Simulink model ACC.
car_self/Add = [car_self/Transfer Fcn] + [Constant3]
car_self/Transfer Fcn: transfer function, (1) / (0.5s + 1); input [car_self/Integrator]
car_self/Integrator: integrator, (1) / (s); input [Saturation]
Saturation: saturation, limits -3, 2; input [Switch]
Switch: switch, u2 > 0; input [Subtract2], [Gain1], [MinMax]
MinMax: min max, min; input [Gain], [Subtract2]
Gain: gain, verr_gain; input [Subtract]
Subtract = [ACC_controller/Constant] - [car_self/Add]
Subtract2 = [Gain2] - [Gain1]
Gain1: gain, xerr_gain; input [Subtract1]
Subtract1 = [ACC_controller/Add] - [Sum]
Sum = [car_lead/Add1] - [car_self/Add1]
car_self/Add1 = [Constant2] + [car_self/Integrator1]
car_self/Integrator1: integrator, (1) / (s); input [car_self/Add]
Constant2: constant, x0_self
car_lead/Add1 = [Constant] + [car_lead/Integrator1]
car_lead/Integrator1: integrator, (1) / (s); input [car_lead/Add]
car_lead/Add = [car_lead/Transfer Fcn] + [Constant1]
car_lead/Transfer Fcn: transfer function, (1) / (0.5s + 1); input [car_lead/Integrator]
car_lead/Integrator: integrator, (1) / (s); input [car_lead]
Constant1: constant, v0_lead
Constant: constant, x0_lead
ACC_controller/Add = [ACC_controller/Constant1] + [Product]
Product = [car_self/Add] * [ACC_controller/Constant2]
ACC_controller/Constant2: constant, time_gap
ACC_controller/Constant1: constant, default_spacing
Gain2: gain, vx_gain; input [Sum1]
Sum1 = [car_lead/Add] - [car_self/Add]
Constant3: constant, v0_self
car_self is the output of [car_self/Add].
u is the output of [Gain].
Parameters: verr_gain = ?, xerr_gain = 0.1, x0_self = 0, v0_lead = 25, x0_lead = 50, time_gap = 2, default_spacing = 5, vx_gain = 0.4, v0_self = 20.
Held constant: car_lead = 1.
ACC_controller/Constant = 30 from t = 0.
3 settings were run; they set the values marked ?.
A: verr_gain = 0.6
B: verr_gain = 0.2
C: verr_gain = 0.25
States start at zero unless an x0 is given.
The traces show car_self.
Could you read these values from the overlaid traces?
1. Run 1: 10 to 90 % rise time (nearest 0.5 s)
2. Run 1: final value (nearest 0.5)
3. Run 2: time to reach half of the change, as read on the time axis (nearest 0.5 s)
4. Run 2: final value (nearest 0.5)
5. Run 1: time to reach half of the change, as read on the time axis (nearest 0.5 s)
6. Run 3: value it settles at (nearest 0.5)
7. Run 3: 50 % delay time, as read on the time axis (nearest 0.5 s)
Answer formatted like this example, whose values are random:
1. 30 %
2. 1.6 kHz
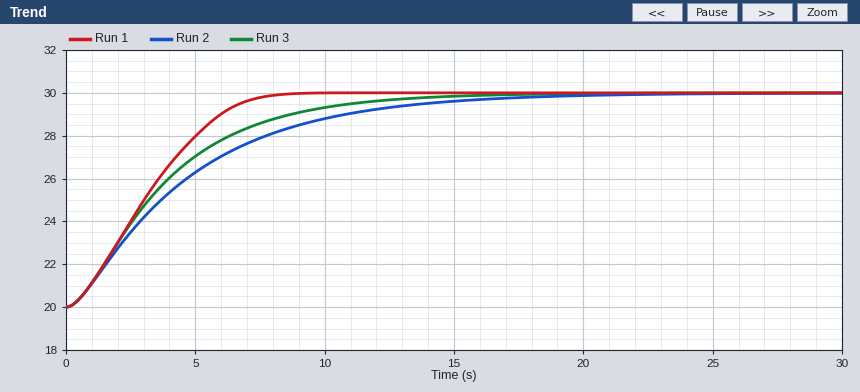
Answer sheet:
1. 5.0 s
2. 30.0
3. 3.5 s
4. 30.0
5. 3.0 s
6. 30.0
7. 3.0 s
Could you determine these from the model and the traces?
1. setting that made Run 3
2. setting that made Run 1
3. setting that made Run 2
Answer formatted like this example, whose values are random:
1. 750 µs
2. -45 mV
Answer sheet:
1. C
2. A
3. B
